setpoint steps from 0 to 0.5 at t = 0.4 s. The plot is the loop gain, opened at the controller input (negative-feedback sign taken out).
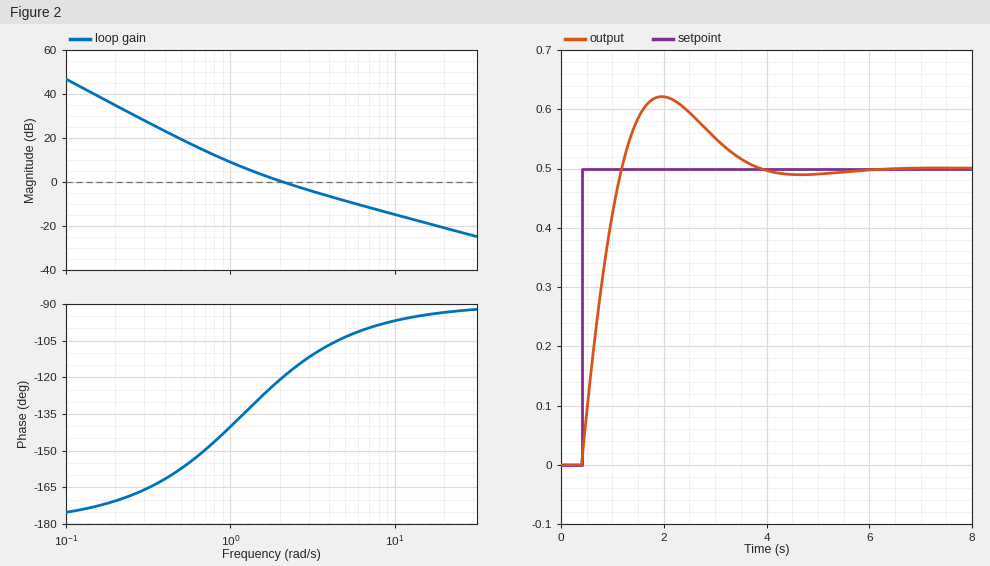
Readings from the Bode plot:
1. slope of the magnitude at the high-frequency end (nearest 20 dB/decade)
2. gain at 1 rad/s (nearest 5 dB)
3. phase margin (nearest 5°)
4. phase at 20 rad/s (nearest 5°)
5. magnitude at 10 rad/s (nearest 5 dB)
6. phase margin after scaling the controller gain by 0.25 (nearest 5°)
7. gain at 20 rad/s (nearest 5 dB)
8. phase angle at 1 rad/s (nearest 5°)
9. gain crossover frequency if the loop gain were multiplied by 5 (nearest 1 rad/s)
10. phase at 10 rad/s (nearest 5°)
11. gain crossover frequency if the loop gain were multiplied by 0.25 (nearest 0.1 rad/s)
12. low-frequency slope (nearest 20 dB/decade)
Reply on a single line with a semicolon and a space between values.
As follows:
-20 dB/decade; 10 dB; 60°; -95°; -15 dB; 35°; -20 dB; -140°; 9 rad/s; -95°; 0.8 rad/s; -40 dB/decade
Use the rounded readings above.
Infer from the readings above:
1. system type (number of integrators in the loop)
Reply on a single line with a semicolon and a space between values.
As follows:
2
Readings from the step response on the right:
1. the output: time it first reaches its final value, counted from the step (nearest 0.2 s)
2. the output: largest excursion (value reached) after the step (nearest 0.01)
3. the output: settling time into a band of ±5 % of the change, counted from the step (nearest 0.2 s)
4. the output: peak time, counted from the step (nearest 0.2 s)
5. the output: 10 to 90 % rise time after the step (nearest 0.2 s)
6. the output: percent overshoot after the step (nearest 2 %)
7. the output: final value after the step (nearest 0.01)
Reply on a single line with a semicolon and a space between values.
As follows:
0.8 s; 0.62; 3.0 s; 1.6 s; 0.6 s; 24 %; 0.50
